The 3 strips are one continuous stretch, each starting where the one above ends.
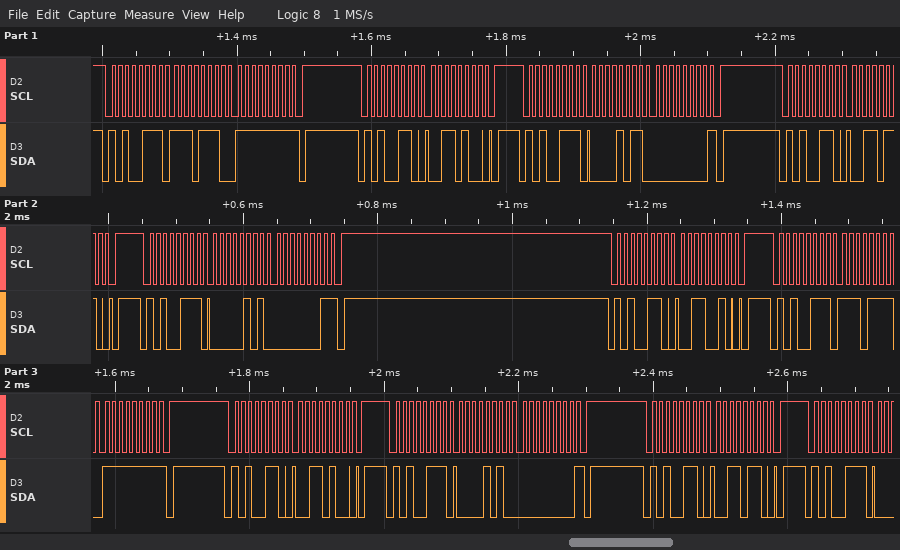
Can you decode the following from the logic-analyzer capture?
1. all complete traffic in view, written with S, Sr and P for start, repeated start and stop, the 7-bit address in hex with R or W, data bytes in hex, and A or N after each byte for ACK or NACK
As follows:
S 53R A EE A FF N P S 53W A 34 A P S 53R A 0B A 00 N P S 53W A 36 A P S 53R A 05 A 01 N P S 53W A 32 A P S 53R A EF A FF N P S 53W A 34 A P S 53R A 0A A 00 N P S 53W A 36 A P S 53R A
